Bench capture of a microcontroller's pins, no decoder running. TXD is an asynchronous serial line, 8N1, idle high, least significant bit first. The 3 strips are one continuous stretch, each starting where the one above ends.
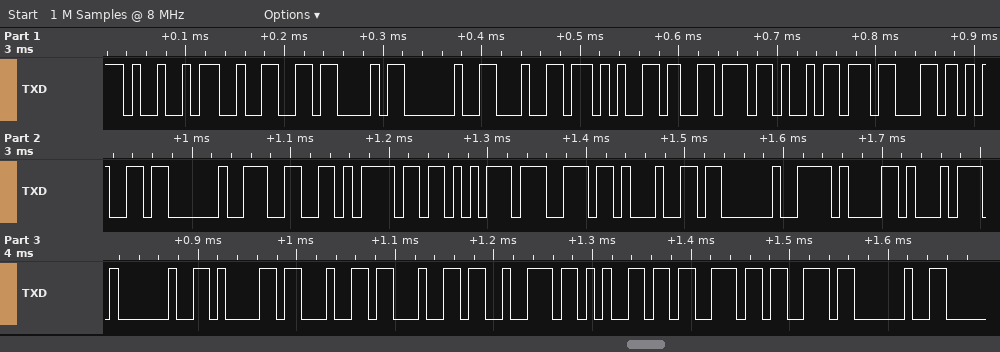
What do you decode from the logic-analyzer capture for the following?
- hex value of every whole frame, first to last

49 32 43 20 64 65 76 69 63 65 20 66 6F 75 6E 64 20 61 74 20 61 64 64 72 65 73 73 20
